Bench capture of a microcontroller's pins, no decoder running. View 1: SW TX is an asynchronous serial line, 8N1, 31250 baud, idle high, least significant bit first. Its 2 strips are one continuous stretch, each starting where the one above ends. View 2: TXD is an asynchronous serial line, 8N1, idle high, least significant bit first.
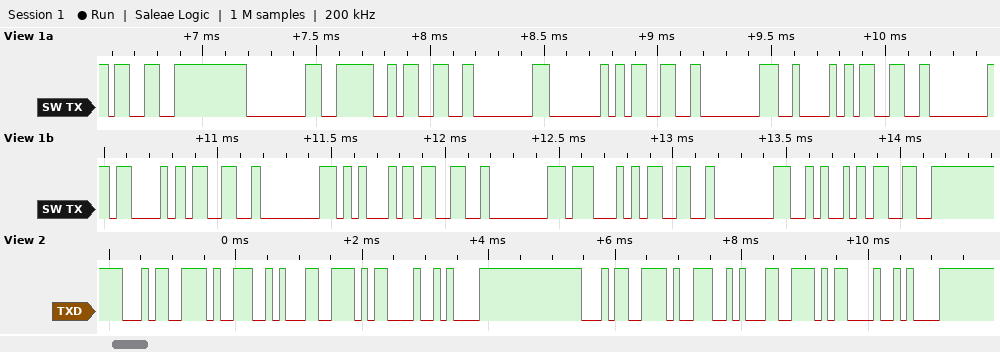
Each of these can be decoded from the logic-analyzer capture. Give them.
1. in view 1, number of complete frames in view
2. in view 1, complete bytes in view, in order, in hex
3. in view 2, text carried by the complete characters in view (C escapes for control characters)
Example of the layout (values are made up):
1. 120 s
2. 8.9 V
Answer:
1. 22
2. 33 80 3E 33 80 40 33 80 42 33 80 43 33 80 45 33 80 47 33 80 4A 33
3. "491\r\n491\r\n"
